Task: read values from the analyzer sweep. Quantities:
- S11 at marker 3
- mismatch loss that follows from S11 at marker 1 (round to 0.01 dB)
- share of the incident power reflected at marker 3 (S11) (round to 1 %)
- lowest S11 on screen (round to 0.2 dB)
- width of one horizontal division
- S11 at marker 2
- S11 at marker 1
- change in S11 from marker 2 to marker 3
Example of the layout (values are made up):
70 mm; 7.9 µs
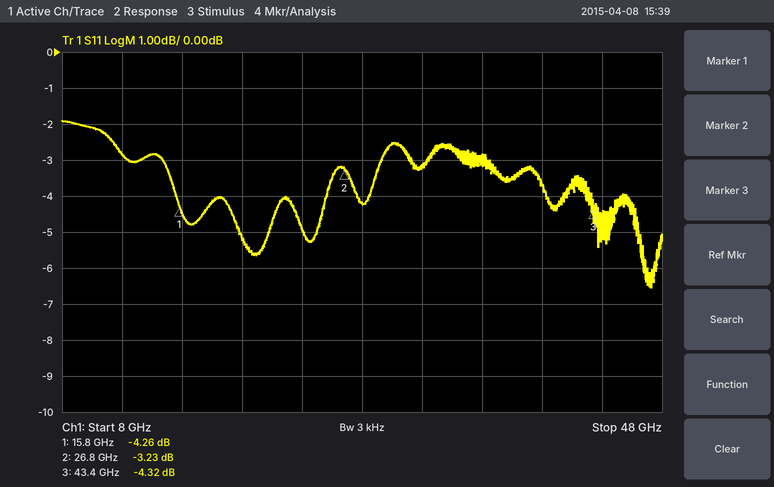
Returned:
-4.32 dB; 2.04 dB; 37 %; -6.6 dB; 4 GHz; -3.23 dB; -4.26 dB; -1.09 dB
